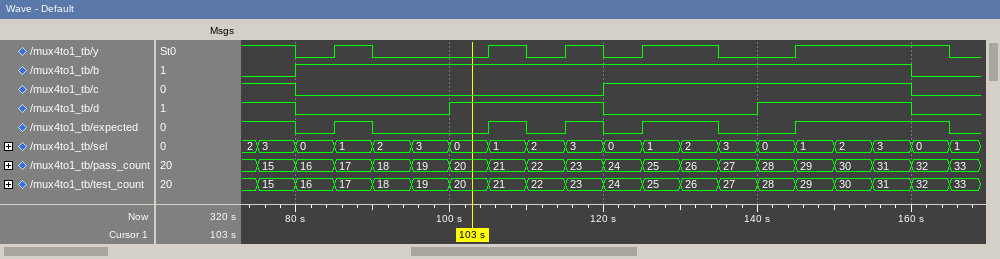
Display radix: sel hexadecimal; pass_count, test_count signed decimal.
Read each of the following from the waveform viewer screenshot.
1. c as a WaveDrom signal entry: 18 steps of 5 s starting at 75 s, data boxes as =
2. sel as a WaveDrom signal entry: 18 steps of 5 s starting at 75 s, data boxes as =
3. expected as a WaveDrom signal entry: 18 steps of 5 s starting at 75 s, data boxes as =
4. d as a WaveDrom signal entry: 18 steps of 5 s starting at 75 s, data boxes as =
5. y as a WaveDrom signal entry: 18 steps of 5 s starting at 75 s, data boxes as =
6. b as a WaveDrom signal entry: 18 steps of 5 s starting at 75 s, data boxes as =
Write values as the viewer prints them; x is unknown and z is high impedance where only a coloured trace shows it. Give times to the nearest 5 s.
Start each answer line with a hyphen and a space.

- {name: 'c', wave: '10.......1.......0'}
- {name: 'sel', wave: '==================', data: '3 0 1 2 3 0 1 2 3 0 1 2 3 0 1 2 3 0'}
- {name: 'expected', wave: '1010..10101.0.1...'}
- {name: 'd', wave: '10...1...0...1...0'}
- {name: 'y', wave: '1010..10101.0.1...'}
- {name: 'b', wave: '01...............0'}
